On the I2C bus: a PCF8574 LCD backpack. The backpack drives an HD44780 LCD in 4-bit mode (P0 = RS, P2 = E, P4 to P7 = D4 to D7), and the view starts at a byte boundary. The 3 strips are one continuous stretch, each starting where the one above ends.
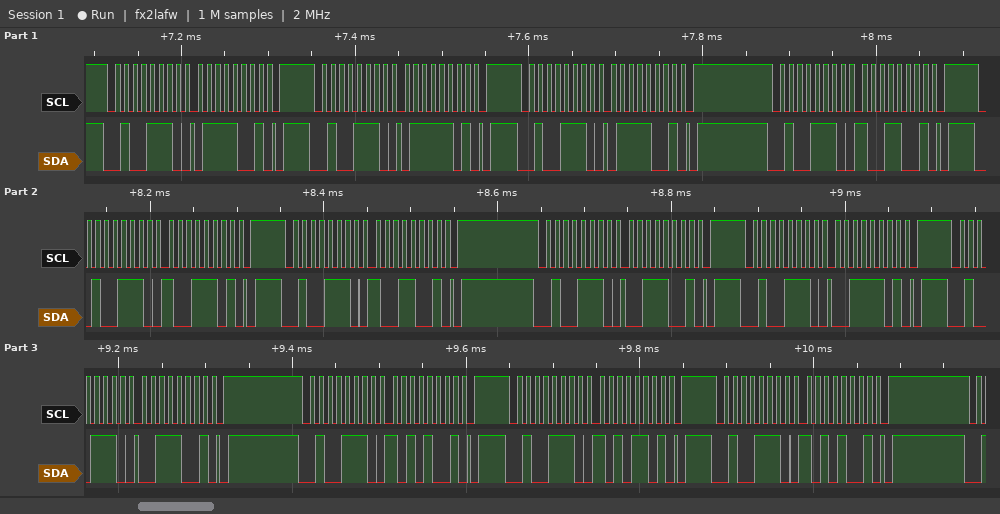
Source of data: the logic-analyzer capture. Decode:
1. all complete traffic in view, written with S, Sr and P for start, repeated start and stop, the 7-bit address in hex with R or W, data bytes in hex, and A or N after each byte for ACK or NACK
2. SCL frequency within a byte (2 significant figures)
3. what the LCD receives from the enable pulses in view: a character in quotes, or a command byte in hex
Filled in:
S 27W A 79 A P S 27W A 7D A P S 27W A 79 A P S 27W A 99 A P S 27W A 9D A P S 27W A 99 A P S 27W A 39 A P S 27W A 3D A P S 27W A 39 A P S 27W A A9 A P S 27W A AD A P S 27W A A9 A P
100 kHz
'y' ':'
